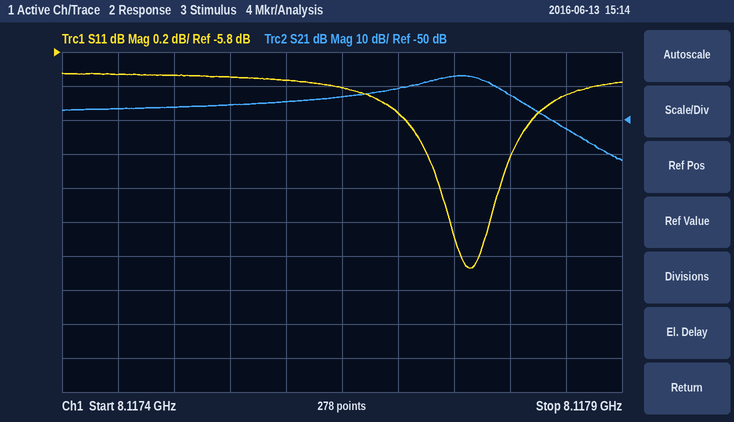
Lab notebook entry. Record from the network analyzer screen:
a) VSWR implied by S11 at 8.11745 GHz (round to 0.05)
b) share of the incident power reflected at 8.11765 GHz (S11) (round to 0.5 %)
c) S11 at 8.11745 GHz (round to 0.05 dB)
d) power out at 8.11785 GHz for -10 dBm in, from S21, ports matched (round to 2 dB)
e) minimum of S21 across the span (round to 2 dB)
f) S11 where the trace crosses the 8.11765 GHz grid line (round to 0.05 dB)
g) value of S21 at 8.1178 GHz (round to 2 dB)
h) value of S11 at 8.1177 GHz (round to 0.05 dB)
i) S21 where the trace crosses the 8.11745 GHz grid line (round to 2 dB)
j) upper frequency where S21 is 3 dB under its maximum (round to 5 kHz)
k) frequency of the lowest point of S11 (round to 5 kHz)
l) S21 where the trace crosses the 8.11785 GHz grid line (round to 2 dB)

3.05
25.0 %
-5.95 dB
-62 dBm
-62 dB
-6.00 dB
-42 dB
-6.15 dB
-46 dB
8.117785 GHz
8.117765 GHz
-52 dB
